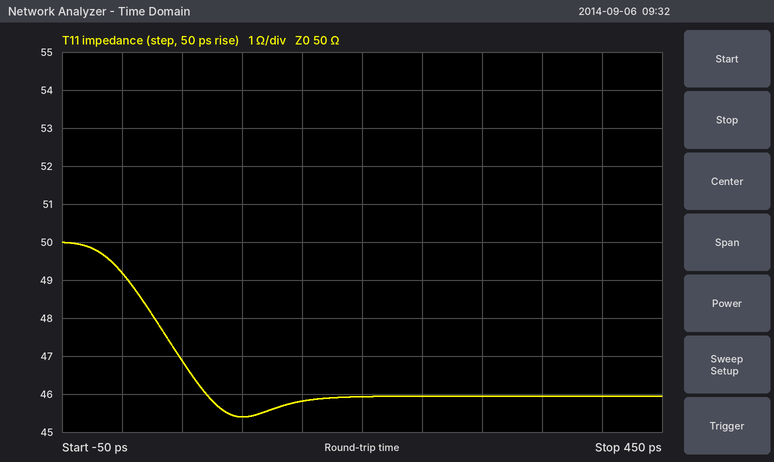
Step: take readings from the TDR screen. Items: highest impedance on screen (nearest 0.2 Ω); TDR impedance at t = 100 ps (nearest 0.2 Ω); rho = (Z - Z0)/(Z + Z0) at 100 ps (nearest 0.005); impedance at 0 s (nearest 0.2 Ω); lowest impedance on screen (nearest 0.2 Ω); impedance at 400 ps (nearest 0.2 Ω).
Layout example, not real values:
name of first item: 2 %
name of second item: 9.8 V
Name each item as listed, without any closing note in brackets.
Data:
highest impedance on screen: 50.0 Ω
TDR impedance at t = 100 ps: 45.4 Ω
rho = (Z - Z0)/(Z + Z0) at 100 ps: -0.050
impedance at 0 s: 49.2 Ω
lowest impedance on screen: 45.4 Ω
impedance at 400 ps: 46.0 Ω
